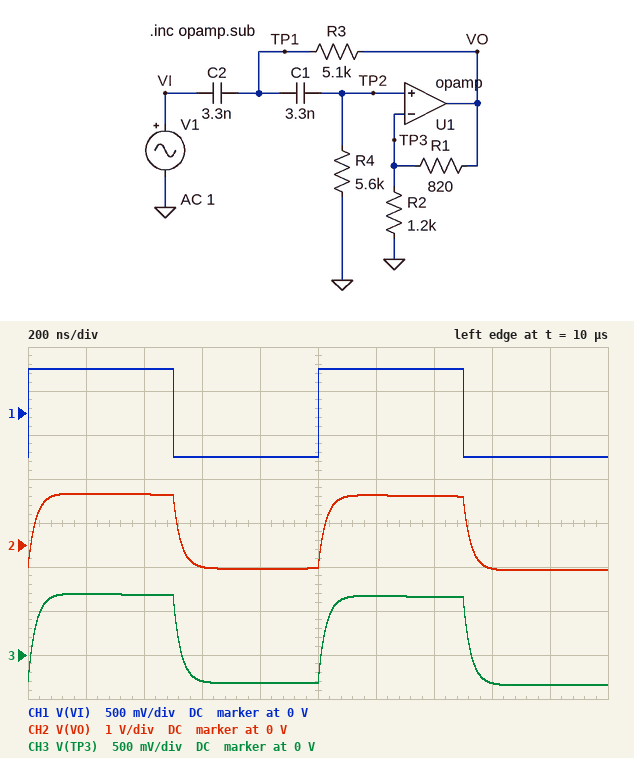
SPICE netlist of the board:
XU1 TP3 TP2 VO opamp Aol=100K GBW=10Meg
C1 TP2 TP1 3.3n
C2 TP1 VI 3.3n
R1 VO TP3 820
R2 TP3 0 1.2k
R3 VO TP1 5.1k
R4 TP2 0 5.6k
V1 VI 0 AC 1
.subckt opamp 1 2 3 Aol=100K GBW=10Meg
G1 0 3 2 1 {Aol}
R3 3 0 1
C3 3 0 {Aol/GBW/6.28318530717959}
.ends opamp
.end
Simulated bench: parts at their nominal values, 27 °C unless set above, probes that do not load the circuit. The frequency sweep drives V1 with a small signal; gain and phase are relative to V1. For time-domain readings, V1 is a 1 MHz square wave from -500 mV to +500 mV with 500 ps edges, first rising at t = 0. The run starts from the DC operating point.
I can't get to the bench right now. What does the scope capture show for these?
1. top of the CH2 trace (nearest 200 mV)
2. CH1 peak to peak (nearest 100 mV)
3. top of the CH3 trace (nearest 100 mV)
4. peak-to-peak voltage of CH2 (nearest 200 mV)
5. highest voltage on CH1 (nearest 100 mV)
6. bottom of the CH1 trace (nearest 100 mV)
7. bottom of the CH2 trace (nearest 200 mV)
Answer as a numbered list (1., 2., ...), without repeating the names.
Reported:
1. 1.2 V
2. 1.0 V
3. 700 mV
4. 1.8 V
5. 500 mV
6. -500 mV
7. -600 mV
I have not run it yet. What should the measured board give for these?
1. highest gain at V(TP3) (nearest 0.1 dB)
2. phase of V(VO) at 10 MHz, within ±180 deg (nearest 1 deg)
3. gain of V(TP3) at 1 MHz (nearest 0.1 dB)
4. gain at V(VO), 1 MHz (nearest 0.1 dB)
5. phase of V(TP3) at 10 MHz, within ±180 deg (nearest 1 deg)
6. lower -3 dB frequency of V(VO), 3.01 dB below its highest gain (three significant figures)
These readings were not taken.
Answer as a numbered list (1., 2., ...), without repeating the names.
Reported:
1. 0.4 dB
2. -59 deg
3. -0.1 dB
4. 4.4 dB
5. -59 deg
6. 8.07 kHz
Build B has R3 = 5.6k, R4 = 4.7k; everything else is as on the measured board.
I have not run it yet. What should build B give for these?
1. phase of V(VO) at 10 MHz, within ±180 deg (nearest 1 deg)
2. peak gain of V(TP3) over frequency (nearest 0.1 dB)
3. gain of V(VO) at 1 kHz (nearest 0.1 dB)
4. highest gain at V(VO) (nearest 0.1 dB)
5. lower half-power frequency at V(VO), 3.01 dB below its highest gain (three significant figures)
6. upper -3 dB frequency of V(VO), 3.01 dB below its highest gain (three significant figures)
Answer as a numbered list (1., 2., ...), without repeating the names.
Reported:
1. -59 deg
2. 0 dB
3. -34.4 dB
4. 4.5 dB
5. 10.4 kHz
6. 5.97 MHz
